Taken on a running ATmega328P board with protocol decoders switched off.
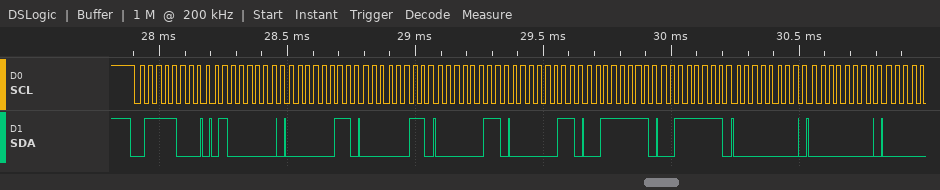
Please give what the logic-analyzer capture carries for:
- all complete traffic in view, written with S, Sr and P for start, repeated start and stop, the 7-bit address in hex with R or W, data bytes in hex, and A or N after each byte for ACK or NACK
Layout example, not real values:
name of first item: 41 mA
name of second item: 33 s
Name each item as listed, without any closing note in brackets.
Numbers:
all complete traffic in view, written with S, Sr and P for start, repeated start and stop, the 7-bit address in hex with R or W, data bytes in hex, and A or N after each byte for ACK or NACK: S 3CW A 40 A 03 A 03 A 03 A 03 A 3F A 3F A 00 A 00 A
